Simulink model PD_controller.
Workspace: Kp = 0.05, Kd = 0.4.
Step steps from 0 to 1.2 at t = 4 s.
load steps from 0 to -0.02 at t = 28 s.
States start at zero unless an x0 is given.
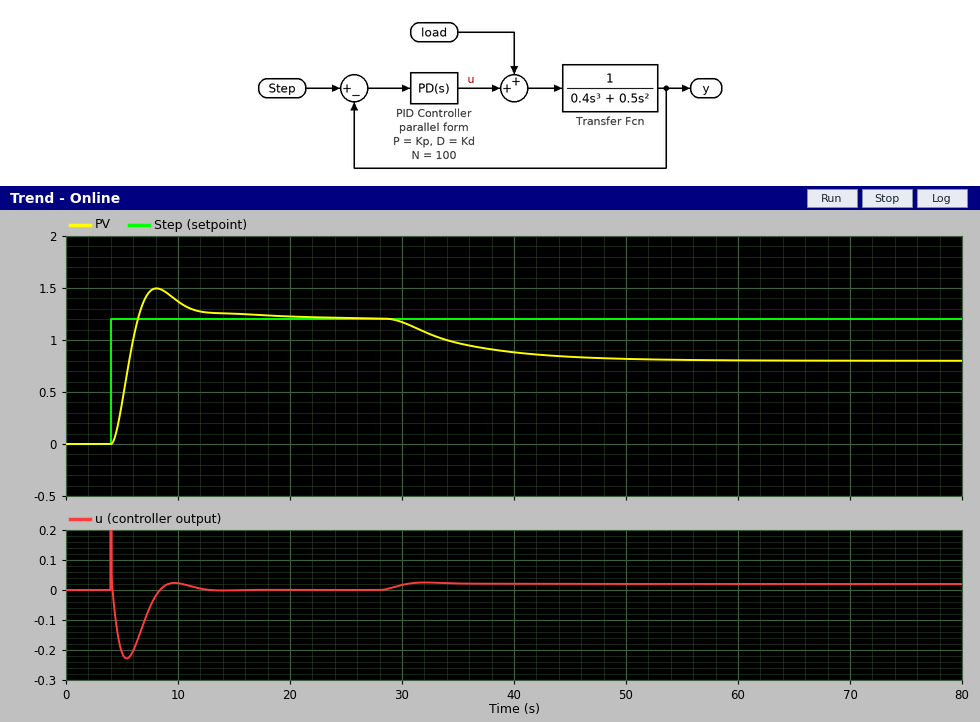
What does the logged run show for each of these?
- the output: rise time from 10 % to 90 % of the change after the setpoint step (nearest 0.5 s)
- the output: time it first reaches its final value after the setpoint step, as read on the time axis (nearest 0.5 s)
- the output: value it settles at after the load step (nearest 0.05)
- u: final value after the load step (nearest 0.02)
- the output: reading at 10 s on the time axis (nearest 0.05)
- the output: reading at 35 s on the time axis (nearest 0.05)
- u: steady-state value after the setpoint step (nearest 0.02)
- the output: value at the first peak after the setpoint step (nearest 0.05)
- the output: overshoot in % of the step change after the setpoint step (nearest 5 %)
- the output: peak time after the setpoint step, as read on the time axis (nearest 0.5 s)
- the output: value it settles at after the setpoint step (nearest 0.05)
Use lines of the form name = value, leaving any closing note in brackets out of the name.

the output: rise time from 10 % to 90 % of the change after the setpoint step = 1.5 s
the output: time it first reaches its final value after the setpoint step, as read on the time axis = 6.5 s
the output: value it settles at after the load step = 0.80
u: final value after the load step = 0.02
the output: reading at 10 s on the time axis = 1.35
the output: reading at 35 s on the time axis = 0.95
u: steady-state value after the setpoint step = 0.00
the output: value at the first peak after the setpoint step = 1.50
the output: overshoot in % of the step change after the setpoint step = 25 %
the output: peak time after the setpoint step, as read on the time axis = 8.0 s
the output: value it settles at after the setpoint step = 1.20
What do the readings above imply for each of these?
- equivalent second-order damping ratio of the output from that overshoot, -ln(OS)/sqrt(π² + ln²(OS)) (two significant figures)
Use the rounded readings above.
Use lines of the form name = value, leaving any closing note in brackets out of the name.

equivalent second-order damping ratio of the output from that overshoot, -ln(OS)/sqrt(π² + ln²(OS)) = 0.40
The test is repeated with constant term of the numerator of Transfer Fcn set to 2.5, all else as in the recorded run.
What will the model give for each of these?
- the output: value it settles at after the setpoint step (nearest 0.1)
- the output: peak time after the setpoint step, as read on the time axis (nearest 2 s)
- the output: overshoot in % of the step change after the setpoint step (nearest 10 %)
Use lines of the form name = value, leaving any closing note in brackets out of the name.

the output: value it settles at after the setpoint step = 1.2
the output: peak time after the setpoint step, as read on the time axis = 6 s
the output: overshoot in % of the step change after the setpoint step = 40 %
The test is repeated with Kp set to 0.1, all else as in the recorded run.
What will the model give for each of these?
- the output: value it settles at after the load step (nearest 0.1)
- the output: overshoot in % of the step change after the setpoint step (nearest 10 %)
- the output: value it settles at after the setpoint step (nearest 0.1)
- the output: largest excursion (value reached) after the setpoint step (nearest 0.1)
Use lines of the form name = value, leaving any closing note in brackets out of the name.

the output: value it settles at after the load step = 1.0
the output: overshoot in % of the step change after the setpoint step = 40 %
the output: value it settles at after the setpoint step = 1.2
the output: largest excursion (value reached) after the setpoint step = 1.7
